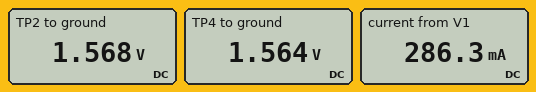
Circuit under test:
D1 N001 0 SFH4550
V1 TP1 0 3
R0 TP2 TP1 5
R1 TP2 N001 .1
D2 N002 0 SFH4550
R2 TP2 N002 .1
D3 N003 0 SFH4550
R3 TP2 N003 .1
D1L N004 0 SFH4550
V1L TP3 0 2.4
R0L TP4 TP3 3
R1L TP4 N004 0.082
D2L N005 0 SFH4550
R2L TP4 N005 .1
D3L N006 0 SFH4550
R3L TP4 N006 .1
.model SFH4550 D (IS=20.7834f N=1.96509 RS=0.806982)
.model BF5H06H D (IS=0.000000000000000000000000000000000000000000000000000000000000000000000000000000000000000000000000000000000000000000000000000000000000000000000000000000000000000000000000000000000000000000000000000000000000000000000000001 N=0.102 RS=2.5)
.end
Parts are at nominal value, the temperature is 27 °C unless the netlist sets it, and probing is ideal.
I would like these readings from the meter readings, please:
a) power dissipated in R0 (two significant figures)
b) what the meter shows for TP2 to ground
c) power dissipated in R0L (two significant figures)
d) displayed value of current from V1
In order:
410 mW
1.568 V
230 mW
286.3 mA
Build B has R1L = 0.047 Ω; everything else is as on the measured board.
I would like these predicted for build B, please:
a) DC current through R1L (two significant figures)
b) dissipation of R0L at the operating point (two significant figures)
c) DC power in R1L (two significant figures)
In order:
95 mA
230 mW
430 µW
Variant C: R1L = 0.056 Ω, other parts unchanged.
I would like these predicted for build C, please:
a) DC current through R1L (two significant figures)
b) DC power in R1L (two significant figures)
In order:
95 mA
500 µW
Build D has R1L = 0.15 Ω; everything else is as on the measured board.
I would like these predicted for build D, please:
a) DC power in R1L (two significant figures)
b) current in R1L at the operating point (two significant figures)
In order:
1.2 mW
91 mA
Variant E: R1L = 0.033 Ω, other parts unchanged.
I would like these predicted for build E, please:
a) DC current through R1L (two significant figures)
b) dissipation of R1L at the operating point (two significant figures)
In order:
96 mA
300 µW
